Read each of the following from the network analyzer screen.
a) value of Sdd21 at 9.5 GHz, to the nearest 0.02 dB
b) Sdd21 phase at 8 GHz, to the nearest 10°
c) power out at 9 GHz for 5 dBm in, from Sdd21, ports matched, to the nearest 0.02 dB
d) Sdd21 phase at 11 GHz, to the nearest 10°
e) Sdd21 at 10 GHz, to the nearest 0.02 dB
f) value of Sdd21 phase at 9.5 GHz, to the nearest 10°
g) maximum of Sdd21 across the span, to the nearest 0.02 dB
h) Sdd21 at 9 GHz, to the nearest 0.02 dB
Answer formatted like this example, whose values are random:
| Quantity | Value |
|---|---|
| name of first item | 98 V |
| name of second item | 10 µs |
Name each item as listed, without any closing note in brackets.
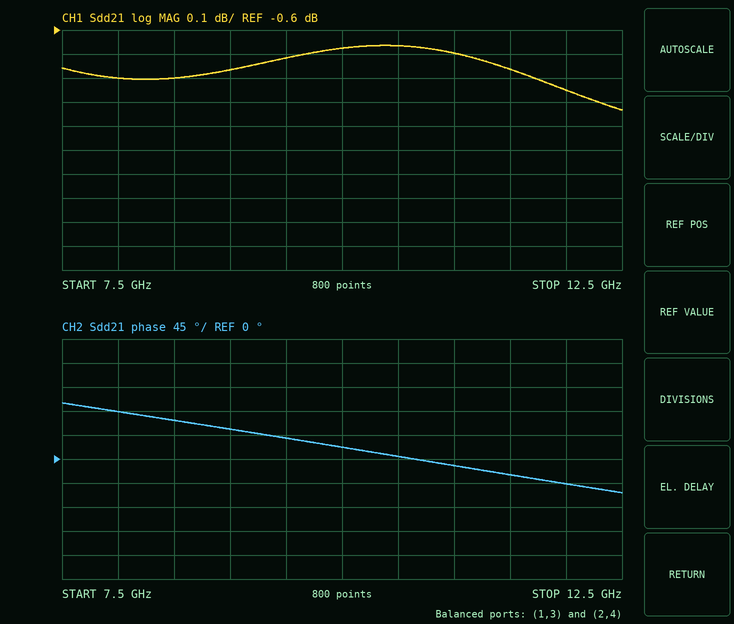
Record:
| Quantity | Value |
|---|---|
| value of Sdd21 at 9.5 GHz, to the nearest 0.02 dB | -0.72 dB |
| Sdd21 phase at 8 GHz, to the nearest 10° | 90° |
| power out at 9 GHz for 5 dBm in, from Sdd21, ports matched, to the nearest 0.02 dB | 4.24 dBm |
| Sdd21 phase at 11 GHz, to the nearest 10° | -10° |
| Sdd21 at 10 GHz, to the nearest 0.02 dB | -0.68 dB |
| value of Sdd21 phase at 9.5 GHz, to the nearest 10° | 40° |
| maximum of Sdd21 across the span, to the nearest 0.02 dB | -0.66 dB |
| Sdd21 at 9 GHz, to the nearest 0.02 dB | -0.76 dB |
